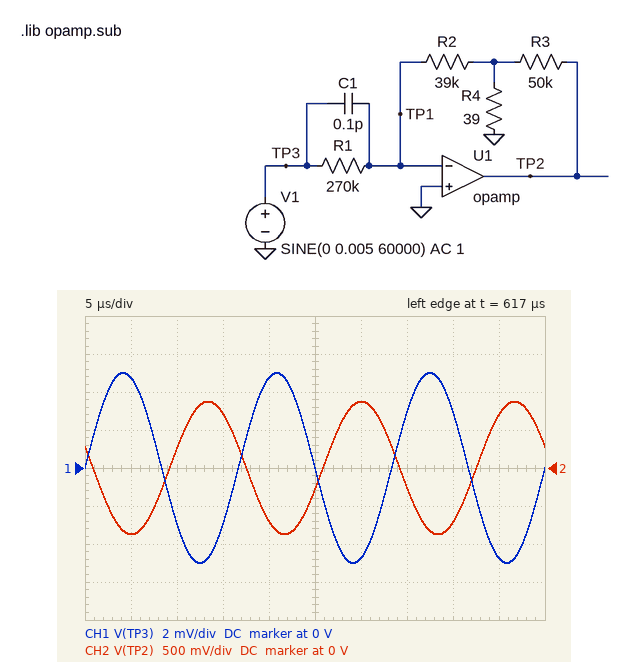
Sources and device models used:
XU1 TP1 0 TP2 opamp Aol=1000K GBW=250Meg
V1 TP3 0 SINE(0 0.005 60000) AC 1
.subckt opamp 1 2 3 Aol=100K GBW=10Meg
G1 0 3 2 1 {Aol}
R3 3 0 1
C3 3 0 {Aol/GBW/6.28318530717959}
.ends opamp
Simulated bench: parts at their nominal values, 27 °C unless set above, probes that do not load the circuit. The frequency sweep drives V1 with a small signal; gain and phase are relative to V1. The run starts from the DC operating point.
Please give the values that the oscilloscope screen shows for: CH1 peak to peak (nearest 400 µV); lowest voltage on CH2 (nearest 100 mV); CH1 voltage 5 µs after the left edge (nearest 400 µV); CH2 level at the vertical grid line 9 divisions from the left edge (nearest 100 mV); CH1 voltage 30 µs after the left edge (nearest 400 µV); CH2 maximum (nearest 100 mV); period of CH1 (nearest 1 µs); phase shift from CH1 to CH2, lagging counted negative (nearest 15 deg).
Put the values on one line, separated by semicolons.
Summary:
10.0 mV; -900 mV; 4.8 mV; 700 mV; -4.8 mV; 900 mV; 17 µs; 165 deg
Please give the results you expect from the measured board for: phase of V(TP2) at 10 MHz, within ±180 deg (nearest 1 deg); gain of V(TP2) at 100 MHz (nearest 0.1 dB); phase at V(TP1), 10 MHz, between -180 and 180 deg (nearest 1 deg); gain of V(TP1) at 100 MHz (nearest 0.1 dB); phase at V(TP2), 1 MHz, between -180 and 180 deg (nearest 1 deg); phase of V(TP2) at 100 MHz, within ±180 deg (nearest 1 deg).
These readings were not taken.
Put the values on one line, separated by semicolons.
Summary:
138 deg; 7.1 dB; 48 deg; -0.8 dB; 108 deg; 112 deg
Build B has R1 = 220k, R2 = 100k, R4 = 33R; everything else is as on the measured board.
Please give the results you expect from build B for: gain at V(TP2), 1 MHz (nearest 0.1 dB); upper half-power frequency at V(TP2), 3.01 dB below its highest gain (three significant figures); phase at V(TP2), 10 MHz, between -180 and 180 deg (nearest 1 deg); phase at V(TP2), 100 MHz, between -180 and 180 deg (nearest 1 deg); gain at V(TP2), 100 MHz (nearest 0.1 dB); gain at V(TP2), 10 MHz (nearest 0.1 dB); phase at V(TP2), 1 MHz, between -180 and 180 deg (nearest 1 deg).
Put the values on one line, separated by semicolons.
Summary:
37.9 dB; 114 kHz; 121 deg; 99 deg; 7.8 dB; 21.8 dB; 102 deg
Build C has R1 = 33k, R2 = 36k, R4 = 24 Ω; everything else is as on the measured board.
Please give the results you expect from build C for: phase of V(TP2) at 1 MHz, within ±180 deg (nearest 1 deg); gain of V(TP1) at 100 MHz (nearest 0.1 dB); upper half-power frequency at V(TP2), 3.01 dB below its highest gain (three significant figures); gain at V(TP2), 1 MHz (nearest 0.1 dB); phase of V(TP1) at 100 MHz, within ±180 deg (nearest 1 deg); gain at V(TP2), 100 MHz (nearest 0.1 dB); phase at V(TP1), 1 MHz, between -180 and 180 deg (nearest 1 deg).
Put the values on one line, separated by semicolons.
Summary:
94 deg; -1.8 dB; 57.6 kHz; 42.3 dB; 17 deg; 6.2 dB; 4 deg
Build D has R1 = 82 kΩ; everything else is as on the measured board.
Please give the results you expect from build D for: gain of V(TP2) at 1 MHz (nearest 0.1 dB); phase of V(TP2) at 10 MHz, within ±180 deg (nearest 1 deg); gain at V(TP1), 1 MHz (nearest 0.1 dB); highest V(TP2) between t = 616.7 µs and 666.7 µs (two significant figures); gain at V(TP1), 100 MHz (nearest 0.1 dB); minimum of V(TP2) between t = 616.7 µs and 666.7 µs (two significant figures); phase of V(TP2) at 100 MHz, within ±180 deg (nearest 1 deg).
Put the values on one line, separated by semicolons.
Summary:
38.1 dB; 109 deg; -9.9 dB; 2.8 V; -1.2 dB; -2.8 V; 110 deg
